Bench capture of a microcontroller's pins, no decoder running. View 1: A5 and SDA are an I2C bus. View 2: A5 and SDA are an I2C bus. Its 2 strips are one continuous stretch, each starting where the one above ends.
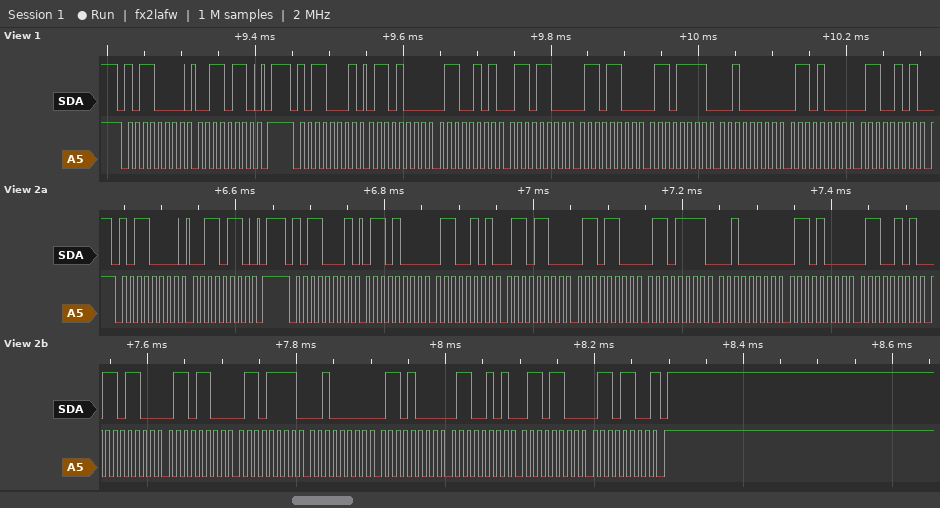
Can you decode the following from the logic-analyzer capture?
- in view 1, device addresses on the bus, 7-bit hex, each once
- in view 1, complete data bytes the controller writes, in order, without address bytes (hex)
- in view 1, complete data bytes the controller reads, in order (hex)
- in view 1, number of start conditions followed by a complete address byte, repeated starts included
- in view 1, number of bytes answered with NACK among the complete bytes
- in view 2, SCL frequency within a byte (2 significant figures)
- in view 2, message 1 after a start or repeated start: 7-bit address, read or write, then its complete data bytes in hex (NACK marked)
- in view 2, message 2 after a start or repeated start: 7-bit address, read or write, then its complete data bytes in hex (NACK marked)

0x58
36
68 65 6C 6C 6F 20 68 65
2
0
100 kHz
0x58 write: 36
0x58 read: 68 65 6C 6C 6F 20 68 65 6C 6C 6F 20 68 65 6C 6C NACK
